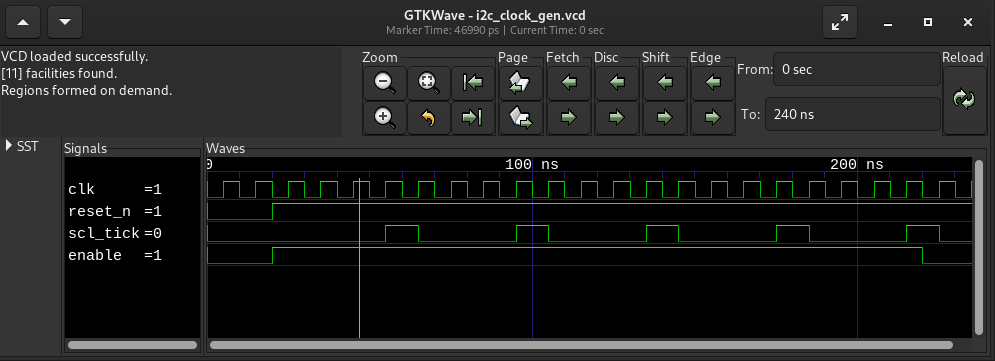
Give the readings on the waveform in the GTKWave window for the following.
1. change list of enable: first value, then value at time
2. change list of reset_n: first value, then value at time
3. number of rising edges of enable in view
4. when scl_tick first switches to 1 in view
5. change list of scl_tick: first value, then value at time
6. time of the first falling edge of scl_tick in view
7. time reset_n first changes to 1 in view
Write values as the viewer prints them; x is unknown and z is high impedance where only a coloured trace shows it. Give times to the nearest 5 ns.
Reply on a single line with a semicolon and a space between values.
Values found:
0, 1 at 20 ns, 0 at 220 ns; 0, 1 at 20 ns; 1; 55 ns; 0, 1 at 55 ns, 0 at 65 ns, 1 at 95 ns, 0 at 105 ns, 1 at 135 ns, 0 at 145 ns, 1 at 175 ns, 0 at 185 ns, 1 at 215 ns, 0 at 225 ns; 65 ns; 20 ns
